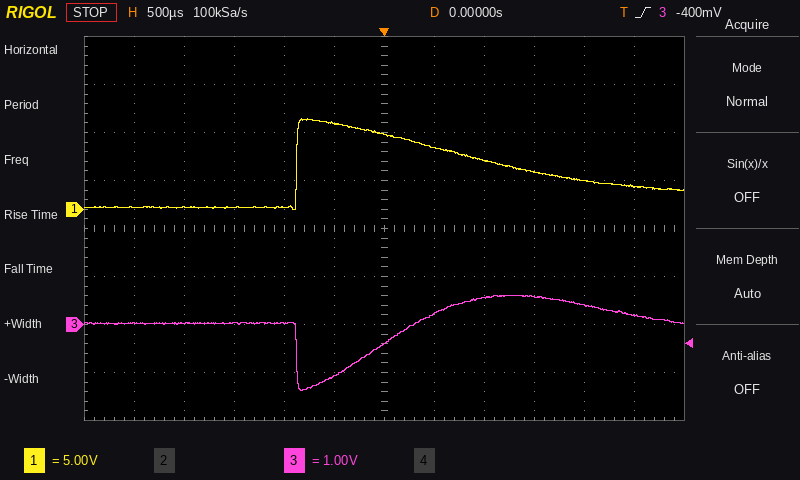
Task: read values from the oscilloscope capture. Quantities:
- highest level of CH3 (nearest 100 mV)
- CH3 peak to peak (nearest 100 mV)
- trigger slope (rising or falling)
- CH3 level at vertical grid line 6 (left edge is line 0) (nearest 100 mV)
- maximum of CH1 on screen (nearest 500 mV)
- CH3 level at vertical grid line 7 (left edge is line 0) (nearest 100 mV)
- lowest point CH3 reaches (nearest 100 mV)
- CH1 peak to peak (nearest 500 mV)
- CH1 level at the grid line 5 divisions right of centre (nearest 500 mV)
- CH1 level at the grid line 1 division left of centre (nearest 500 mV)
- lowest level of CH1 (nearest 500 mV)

600 mV
2.0 V
rising
-400 mV
9.5 V
200 mV
-1.4 V
9.5 V
2.5 V
9.0 V
0.0 V
